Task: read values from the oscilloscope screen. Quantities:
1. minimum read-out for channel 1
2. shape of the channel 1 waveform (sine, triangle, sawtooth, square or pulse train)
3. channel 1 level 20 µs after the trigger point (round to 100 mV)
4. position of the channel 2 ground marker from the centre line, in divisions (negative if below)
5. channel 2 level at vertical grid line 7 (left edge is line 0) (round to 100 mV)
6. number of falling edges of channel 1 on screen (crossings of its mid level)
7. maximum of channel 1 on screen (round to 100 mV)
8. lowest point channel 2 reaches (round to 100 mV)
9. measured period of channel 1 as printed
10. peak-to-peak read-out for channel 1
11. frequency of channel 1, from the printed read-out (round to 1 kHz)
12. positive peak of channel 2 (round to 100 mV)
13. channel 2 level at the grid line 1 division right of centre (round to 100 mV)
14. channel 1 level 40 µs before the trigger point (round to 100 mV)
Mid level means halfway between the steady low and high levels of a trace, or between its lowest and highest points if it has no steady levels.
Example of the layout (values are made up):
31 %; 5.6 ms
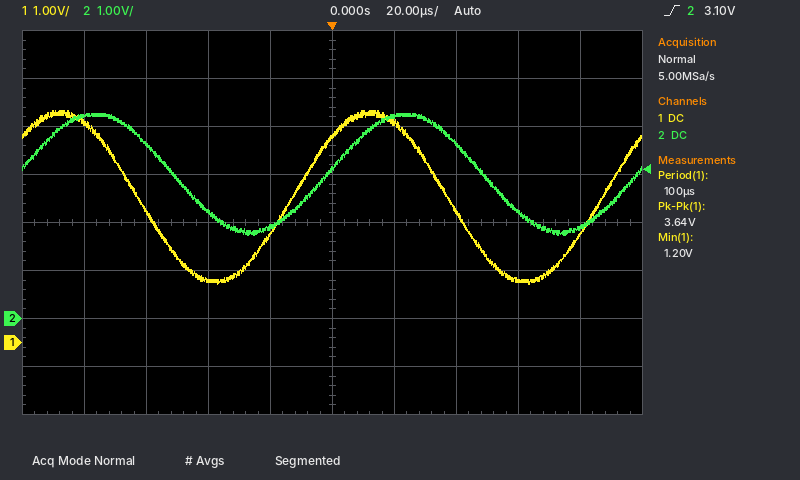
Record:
1.20 V; sine; 4.6 V; -2.0 div; 3.6 V; 2; 4.8 V; 1.7 V; 100 µs; 3.64 V; 10 kHz; 4.3 V; 4.2 V; 1.3 V
